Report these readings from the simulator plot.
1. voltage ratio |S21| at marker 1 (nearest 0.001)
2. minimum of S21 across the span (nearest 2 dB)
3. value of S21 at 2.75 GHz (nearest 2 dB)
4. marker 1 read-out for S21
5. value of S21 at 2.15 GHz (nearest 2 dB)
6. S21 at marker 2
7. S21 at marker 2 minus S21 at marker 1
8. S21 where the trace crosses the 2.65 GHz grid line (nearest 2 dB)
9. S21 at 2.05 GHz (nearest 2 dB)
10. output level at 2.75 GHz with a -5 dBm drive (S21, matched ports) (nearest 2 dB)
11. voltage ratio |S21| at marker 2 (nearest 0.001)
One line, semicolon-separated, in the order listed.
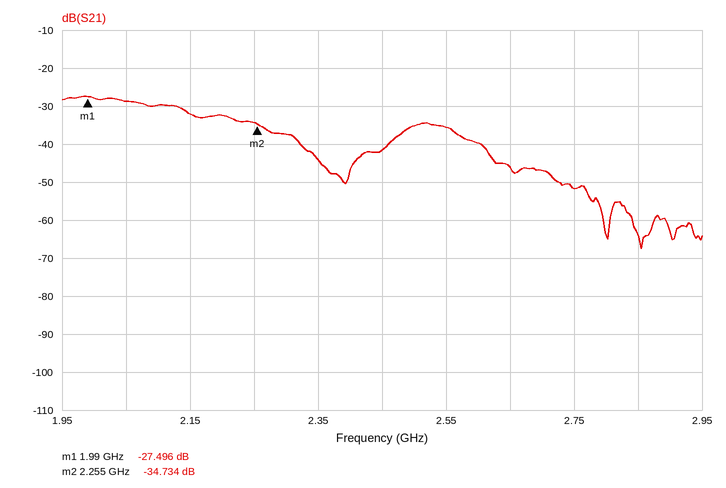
0.042; -68 dB; -52 dB; -27.496 dB; -32 dB; -34.734 dB; -7.238 dB; -46 dB; -28 dB; -56 dBm; 0.018
